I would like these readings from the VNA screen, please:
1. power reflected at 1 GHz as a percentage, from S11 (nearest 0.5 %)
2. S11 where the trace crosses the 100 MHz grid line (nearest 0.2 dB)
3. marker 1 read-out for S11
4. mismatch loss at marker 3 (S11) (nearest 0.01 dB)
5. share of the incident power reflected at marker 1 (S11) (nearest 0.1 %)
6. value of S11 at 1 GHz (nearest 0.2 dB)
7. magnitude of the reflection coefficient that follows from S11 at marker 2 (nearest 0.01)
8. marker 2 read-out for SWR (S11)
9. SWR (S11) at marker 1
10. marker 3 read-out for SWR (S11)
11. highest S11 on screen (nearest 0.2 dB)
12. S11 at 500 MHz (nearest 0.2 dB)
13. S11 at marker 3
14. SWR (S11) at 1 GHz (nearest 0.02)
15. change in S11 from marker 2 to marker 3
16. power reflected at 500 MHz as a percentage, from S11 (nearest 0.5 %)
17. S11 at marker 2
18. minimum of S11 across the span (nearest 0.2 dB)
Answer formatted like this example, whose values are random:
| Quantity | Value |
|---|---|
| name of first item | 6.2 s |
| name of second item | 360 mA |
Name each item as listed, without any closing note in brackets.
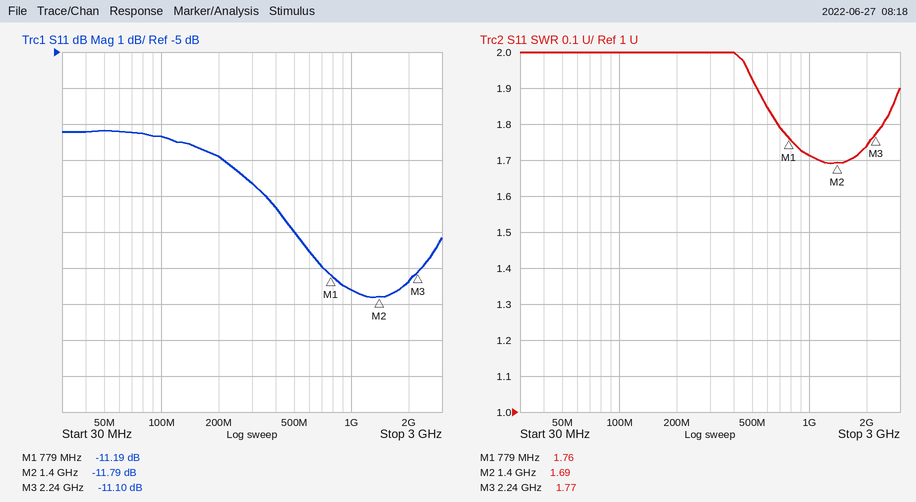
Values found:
| Quantity | Value |
|---|---|
| power reflected at 1 GHz as a percentage, from S11 | 7.0 % |
| S11 where the trace crosses the 100 MHz grid line | -7.4 dB |
| marker 1 read-out for S11 | -11.19 dB |
| mismatch loss at marker 3 (S11) | 0.35 dB |
| share of the incident power reflected at marker 1 (S11) | 7.6 % |
| value of S11 at 1 GHz | -11.6 dB |
| magnitude of the reflection coefficient that follows from S11 at marker 2 | 0.26 |
| marker 2 read-out for SWR | 1.69 |
| SWR (S11) at marker 1 | 1.76 |
| marker 3 read-out for SWR | 1.77 |
| highest S11 on screen | -7.2 dB |
| S11 at 500 MHz | -10.0 dB |
| S11 at marker 3 | -11.10 dB |
| SWR (S11) at 1 GHz | 1.72 |
| change in S11 from marker 2 to marker 3 | 0.69 dB |
| power reflected at 500 MHz as a percentage, from S11 | 10.0 % |
| S11 at marker 2 | -11.79 dB |
| minimum of S11 across the span | -11.8 dB |
